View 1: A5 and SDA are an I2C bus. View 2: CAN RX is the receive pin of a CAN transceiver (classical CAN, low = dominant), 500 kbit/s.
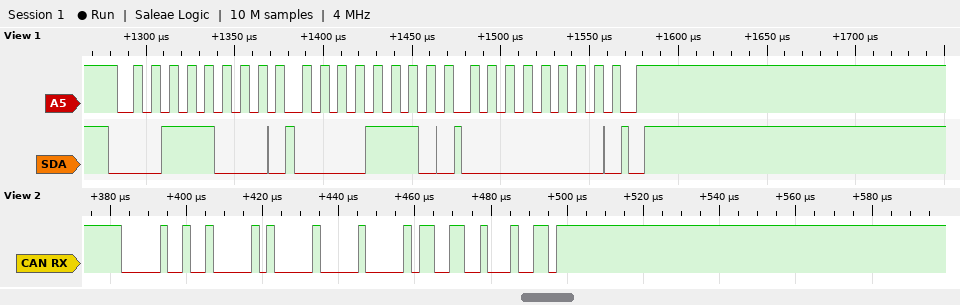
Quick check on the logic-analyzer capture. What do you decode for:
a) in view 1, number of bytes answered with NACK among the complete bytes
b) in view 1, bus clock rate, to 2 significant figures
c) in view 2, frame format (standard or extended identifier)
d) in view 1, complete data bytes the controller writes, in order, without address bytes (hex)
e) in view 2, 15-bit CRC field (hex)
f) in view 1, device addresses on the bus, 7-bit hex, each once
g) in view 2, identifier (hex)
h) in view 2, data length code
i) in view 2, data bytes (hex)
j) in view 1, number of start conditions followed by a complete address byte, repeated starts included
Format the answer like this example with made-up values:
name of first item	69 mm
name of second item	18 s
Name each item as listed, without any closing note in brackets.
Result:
in view 1, number of bytes answered with NACK among the complete bytes	0
in view 1, bus clock rate, to 2 significant figures	100 kHz
in view 2, frame format	standard
in view 1, complete data bytes the controller writes, in order, without address bytes	0E 00
in view 2, 15-bit CRC field	0x4C89
in view 1, device addresses on the bus, 7-bit hex, each once	0x1C
in view 2, identifier	0x012
in view 2, data length code	2
in view 2, data bytes	00 01
in view 1, number of start conditions followed by a complete address byte, repeated starts included	1
